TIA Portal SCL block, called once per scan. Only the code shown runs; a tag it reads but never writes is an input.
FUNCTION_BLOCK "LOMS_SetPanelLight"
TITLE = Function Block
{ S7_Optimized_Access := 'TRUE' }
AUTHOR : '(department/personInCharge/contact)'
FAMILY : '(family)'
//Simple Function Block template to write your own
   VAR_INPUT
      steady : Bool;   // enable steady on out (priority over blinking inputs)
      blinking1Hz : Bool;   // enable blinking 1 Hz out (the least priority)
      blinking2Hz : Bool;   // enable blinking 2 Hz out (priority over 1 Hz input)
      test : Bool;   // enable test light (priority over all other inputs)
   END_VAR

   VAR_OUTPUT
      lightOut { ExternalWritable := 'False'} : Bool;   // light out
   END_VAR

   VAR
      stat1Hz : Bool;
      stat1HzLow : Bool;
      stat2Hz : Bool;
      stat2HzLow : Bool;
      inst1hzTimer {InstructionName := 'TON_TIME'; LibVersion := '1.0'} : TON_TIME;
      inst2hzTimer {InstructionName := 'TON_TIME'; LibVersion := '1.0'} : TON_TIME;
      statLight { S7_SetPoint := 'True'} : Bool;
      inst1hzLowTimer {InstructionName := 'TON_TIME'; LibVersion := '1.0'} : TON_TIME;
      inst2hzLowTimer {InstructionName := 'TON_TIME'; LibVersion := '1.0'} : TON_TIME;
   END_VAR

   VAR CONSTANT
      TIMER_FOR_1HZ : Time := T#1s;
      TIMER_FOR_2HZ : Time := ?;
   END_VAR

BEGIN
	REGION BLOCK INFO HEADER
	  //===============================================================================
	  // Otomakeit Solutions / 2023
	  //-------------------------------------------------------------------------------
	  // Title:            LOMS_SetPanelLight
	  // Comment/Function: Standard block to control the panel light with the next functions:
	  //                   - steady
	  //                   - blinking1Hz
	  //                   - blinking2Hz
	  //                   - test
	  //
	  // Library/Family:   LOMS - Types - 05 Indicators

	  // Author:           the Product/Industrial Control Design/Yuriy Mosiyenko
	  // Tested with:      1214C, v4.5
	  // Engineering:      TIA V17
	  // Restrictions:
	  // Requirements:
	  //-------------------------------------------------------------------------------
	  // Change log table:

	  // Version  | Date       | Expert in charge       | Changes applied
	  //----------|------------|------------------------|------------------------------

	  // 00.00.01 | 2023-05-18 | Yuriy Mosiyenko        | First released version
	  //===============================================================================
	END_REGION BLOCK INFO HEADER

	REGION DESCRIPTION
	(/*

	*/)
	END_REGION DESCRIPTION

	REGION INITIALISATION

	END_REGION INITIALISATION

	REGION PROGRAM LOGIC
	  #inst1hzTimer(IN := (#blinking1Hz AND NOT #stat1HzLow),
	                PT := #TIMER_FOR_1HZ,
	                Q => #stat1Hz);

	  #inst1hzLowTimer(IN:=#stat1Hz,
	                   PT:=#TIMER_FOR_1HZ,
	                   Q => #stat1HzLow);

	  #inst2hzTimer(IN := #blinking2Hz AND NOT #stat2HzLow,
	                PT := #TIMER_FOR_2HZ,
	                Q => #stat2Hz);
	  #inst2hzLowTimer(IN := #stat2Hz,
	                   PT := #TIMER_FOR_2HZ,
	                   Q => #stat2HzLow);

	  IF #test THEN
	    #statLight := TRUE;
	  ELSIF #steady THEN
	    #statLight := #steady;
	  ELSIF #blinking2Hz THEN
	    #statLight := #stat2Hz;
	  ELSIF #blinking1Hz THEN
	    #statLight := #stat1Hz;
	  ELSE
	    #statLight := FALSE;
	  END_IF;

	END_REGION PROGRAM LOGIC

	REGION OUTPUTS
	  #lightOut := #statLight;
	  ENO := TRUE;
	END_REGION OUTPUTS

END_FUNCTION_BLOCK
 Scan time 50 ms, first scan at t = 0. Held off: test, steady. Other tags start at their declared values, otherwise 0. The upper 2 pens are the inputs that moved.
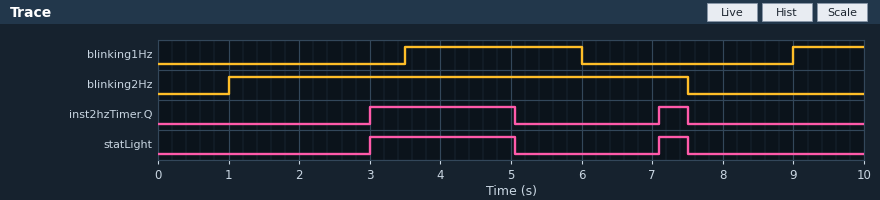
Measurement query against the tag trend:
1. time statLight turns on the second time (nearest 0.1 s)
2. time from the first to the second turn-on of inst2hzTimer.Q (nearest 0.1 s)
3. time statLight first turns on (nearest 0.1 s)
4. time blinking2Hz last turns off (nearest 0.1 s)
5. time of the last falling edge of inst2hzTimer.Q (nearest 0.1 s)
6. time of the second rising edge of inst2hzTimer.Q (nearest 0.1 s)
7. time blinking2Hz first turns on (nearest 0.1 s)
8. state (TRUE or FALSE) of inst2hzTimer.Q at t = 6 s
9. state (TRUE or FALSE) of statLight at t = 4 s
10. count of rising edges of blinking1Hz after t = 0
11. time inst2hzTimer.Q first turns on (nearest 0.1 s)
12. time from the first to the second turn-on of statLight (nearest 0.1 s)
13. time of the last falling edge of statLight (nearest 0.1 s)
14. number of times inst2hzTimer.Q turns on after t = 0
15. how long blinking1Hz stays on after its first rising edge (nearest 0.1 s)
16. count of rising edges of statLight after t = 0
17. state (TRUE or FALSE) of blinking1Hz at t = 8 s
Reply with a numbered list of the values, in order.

1. 7.1 s
2. 4.1 s
3. 3.0 s
4. 7.5 s
5. 7.5 s
6. 7.1 s
7. 1.0 s
8. FALSE
9. TRUE
10. 2
11. 3.0 s
12. 4.1 s
13. 7.5 s
14. 2
15. 2.5 s
16. 2
17. FALSE
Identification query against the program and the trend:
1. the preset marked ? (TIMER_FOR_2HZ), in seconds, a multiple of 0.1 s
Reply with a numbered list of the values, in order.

1. 2.0 s
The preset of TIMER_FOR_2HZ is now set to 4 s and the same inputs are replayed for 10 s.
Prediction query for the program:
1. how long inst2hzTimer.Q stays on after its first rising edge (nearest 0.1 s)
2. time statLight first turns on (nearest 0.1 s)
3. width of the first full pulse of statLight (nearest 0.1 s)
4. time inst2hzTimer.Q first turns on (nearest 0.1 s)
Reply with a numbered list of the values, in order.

1. 2.5 s
2. 5.0 s
3. 2.5 s
4. 5.0 s
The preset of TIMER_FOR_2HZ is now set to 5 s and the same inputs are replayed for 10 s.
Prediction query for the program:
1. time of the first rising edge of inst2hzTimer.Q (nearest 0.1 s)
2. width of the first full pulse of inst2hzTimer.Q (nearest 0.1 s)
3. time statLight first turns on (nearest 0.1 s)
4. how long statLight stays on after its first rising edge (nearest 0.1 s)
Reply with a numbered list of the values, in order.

1. 6.0 s
2. 1.5 s
3. 6.0 s
4. 1.5 s
